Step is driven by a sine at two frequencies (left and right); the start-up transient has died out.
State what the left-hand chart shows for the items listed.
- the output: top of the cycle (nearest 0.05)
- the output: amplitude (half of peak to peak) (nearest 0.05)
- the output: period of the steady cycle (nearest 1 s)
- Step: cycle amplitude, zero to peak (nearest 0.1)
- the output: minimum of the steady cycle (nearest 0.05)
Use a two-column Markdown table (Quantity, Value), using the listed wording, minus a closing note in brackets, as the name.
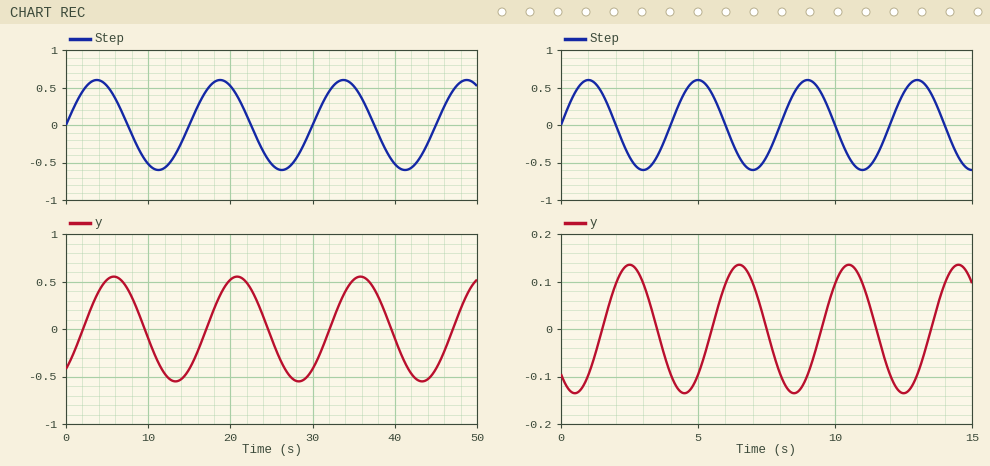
| Quantity | Value |
|---|---|
| the output: top of the cycle | 0.55 |
| the output: amplitude (half of peak to peak) | 0.55 |
| the output: period of the steady cycle | 15 s |
| Step: cycle amplitude, zero to peak | 0.6 |
| the output: minimum of the steady cycle | -0.55 |
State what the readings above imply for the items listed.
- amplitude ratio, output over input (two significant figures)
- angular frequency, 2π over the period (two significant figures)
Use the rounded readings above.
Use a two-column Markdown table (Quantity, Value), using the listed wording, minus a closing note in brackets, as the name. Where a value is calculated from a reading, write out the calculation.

| Quantity | Value |
|---|---|
| amplitude ratio, output over input | 0.55 / 0.6 = 0.92 |
| angular frequency, 2π over the period | 2π / 15 = 0.42 rad/s |
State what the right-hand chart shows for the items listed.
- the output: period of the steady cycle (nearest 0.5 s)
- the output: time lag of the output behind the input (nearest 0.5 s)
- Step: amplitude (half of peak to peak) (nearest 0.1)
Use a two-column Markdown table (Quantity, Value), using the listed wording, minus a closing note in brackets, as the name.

| Quantity | Value |
|---|---|
| the output: period of the steady cycle | 4.0 s |
| the output: time lag of the output behind the input | 1.5 s |
| Step: amplitude (half of peak to peak) | 0.6 |
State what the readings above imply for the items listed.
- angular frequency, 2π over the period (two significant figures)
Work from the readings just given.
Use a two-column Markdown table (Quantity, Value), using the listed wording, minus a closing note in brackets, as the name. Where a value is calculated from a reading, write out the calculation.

| Quantity | Value |
|---|---|
| angular frequency, 2π over the period | 2π / 4 = 1.6 rad/s |
